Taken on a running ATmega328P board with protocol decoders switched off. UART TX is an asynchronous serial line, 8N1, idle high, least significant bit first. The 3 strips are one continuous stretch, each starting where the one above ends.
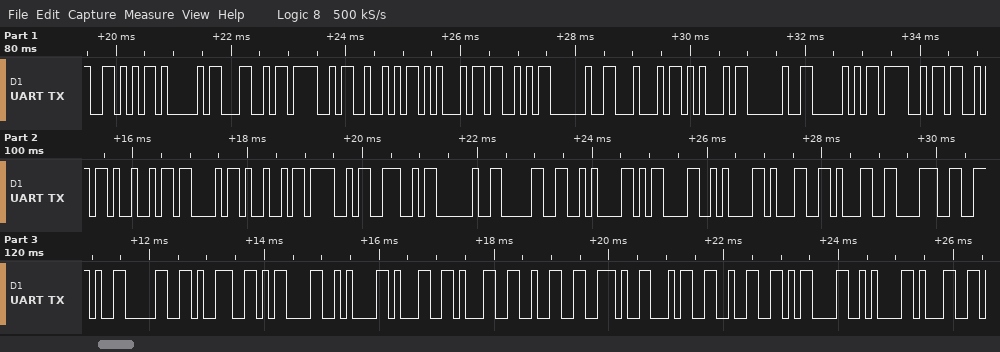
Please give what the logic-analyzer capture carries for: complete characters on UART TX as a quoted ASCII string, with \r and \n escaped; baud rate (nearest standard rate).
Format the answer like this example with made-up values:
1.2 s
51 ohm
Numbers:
"VALORES DE POSICION 0\n\r\n118.09\r\n112.42\r\n1"
9600 baud
